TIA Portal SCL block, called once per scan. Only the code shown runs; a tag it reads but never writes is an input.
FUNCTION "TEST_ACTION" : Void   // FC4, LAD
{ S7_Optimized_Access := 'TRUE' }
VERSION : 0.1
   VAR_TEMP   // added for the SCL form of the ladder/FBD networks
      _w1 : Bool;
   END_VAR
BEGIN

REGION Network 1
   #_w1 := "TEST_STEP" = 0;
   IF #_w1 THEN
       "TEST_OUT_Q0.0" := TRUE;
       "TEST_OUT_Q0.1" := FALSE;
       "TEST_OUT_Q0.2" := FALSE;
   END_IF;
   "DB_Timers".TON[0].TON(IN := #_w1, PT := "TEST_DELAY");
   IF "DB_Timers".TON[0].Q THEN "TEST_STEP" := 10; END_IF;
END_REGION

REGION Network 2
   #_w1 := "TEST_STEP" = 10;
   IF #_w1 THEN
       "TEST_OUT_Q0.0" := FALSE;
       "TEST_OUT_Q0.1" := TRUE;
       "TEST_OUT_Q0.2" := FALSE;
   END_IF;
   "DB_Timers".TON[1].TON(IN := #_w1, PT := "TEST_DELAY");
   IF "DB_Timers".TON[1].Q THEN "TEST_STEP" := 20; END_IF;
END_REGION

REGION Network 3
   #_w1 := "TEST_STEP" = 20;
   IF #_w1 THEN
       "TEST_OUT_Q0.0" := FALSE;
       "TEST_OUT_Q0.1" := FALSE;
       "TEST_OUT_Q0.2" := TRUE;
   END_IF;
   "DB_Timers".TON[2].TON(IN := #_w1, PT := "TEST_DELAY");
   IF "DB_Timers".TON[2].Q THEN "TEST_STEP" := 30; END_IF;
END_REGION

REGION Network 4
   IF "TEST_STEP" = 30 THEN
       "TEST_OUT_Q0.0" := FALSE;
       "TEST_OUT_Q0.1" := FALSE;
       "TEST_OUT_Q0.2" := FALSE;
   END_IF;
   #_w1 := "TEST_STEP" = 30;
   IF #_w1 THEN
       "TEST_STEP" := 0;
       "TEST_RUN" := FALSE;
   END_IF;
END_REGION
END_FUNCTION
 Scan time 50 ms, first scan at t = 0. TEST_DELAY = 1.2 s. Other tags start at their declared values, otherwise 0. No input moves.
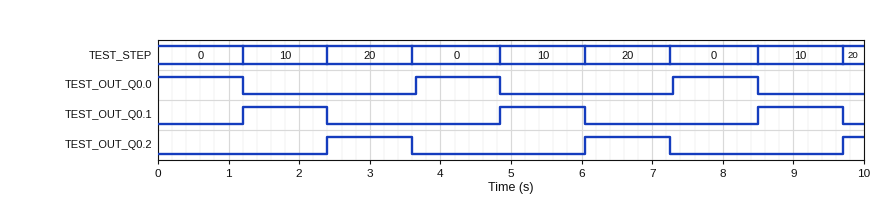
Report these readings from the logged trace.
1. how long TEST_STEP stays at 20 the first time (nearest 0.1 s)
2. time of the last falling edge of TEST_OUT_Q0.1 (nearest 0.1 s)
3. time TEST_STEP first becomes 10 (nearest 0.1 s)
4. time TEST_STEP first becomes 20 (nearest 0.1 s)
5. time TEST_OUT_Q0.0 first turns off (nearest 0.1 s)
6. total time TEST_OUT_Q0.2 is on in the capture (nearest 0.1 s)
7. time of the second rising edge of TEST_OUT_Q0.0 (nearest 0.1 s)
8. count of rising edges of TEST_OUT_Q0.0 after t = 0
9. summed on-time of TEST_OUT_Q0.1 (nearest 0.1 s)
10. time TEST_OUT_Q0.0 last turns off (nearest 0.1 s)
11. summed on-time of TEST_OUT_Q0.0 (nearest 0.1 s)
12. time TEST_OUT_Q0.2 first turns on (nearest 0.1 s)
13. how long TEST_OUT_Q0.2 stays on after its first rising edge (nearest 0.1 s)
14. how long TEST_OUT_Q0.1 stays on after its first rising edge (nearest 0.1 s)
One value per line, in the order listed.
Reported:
1.2 s
9.7 s
1.2 s
2.4 s
1.2 s
2.7 s
7.3 s
2
3.6 s
8.5 s
3.6 s
2.4 s
1.2 s
1.2 s
